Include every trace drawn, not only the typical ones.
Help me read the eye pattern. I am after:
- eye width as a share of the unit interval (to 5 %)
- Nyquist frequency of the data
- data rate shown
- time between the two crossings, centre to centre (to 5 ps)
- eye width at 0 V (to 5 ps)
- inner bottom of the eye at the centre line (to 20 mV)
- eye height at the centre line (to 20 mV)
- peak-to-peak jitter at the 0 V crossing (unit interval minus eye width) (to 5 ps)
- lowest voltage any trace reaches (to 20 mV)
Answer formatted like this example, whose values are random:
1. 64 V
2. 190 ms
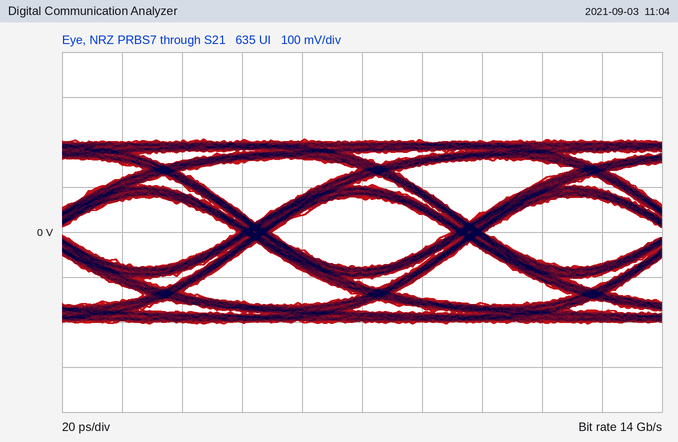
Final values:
1. 85 %
2. 7 GHz
3. 14 Gb/s
4. 70 ps
5. 60 ps
6. -80 mV
7. 160 mV
8. 10 ps
9. -200 mV
